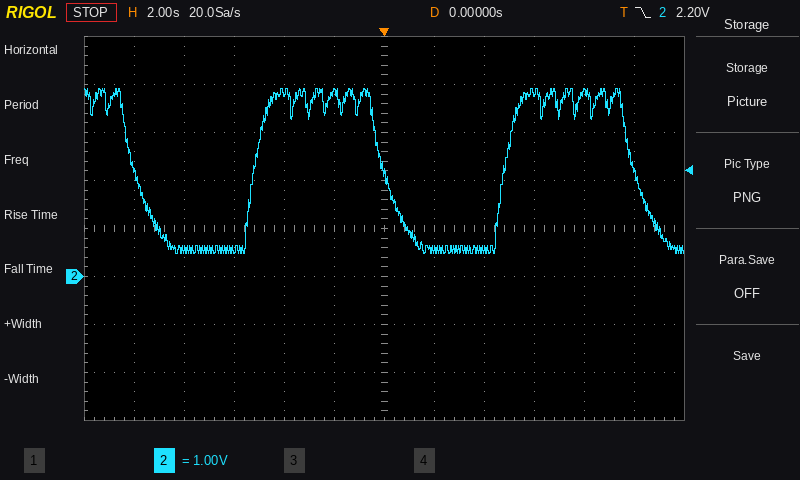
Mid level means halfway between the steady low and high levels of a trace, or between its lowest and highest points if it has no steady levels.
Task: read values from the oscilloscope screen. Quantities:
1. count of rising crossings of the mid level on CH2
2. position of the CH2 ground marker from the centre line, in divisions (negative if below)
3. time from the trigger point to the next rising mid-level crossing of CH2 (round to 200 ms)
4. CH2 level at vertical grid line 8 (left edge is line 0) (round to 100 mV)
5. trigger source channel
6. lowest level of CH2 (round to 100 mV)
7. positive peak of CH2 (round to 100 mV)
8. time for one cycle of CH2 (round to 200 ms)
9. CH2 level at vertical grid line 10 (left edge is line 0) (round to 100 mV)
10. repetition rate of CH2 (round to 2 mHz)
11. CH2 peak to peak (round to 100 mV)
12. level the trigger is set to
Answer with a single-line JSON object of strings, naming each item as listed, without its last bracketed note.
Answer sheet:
{"count of rising crossings of the mid level on CH2": "2", "position of the CH2 ground marker from the centre line, in divisions": "-1.0 div", "time from the trigger point to the next rising mid-level crossing of CH2": "4.8 s", "CH2 level at vertical grid line 8 (left edge is line 0)": "600 mV", "trigger source channel": "CH2", "lowest level of CH2": "500 mV", "positive peak of CH2": "3.9 V", "time for one cycle of CH2": "10.0 s", "CH2 level at vertical grid line 10 (left edge is line 0)": "3.8 V", "repetition rate of CH2": "100 mHz", "CH2 peak to peak": "3.4 V", "level the trigger is set to": "2.20 V"}
